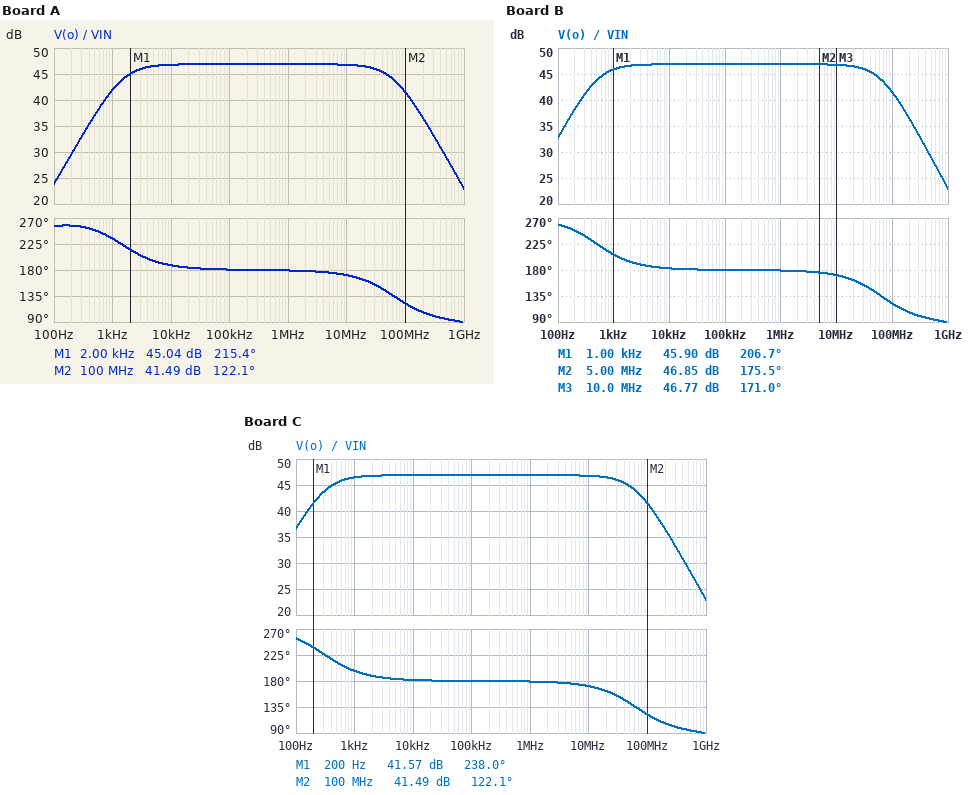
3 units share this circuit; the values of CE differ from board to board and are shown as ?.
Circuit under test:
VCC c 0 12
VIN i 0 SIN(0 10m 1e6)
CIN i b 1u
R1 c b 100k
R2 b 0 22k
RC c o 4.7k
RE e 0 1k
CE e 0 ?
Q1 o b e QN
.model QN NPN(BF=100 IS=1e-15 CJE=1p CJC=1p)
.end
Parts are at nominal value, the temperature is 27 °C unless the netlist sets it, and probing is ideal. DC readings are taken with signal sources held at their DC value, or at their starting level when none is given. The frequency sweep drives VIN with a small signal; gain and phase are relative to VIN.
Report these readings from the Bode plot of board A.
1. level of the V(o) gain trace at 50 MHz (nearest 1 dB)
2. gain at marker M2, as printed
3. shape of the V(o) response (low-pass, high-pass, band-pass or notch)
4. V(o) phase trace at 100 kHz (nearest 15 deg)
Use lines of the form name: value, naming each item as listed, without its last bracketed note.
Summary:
level of the V(o) gain trace at 50 MHz: 45 dB
gain at marker M2, as printed: 41.49 dB
shape of the V(o) response: band-pass
V(o) phase trace at 100 kHz: 180 deg
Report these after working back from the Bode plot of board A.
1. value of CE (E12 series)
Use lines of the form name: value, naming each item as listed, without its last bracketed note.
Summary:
value of CE: 5.6 µF
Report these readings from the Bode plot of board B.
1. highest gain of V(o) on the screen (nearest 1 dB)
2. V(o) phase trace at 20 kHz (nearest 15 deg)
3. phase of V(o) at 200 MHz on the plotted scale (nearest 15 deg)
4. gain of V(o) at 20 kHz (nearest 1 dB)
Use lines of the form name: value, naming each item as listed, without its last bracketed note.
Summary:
highest gain of V(o) on the screen: 47 dB
V(o) phase trace at 20 kHz: 180 deg
phase of V(o) at 200 MHz on the plotted scale: 105 deg
gain of V(o) at 20 kHz: 47 dB
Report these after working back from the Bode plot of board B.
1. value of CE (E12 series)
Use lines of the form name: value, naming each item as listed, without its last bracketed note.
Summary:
value of CE: 18 µF
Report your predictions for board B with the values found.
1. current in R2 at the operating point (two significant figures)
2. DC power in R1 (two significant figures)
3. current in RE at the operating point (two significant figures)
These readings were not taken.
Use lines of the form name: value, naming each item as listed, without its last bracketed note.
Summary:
current in R2 at the operating point: 88 µA
DC power in R1: 1.0 mW
current in RE at the operating point: 1.2 mA
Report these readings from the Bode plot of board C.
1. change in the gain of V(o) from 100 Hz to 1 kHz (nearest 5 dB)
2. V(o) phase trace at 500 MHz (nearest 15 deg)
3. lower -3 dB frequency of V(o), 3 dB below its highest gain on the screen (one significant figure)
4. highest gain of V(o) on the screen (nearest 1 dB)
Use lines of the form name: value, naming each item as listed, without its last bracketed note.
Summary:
change in the gain of V(o) from 100 Hz to 1 kHz: 10 dB
V(o) phase trace at 500 MHz: 90 deg
lower -3 dB frequency of V(o), 3 dB below its highest gain on the screen: 300 Hz
highest gain of V(o) on the screen: 47 dB
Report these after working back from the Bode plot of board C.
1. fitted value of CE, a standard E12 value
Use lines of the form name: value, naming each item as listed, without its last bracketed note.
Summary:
fitted value of CE, a standard E12 value: 33 µF
